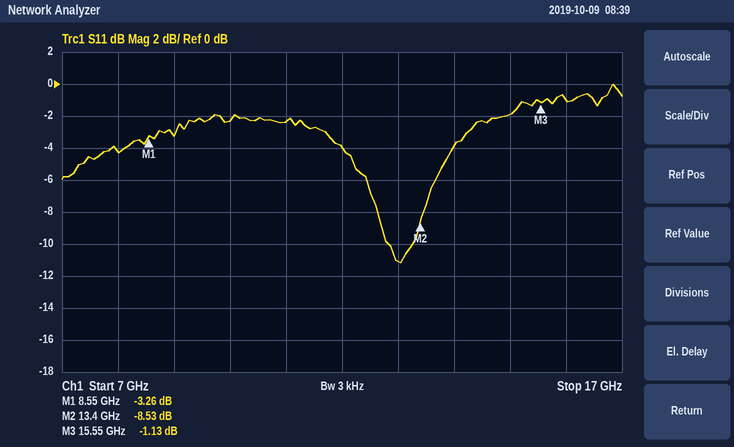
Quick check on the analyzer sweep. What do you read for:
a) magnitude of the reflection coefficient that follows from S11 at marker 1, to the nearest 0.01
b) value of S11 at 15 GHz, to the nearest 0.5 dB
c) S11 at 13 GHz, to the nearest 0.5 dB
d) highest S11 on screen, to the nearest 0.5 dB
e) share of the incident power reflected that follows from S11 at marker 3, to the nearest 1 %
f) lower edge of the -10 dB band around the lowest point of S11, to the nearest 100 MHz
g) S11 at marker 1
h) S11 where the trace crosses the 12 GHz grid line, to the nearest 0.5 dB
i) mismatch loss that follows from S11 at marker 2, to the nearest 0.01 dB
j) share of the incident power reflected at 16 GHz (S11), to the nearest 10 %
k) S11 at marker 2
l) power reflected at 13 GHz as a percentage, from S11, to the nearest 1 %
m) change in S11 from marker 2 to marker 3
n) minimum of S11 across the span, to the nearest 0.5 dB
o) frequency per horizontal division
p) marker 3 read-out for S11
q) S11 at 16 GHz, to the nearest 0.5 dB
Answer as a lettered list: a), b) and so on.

a) 0.69
b) -2.0 dB
c) -11.0 dB
d) 0.0 dB
e) 77 %
f) 12.8 GHz
g) -3.26 dB
h) -4.0 dB
i) 0.66 dB
j) 80 %
k) -8.53 dB
l) 8 %
m) 7.40 dB
n) -11.0 dB
o) 1 GHz
p) -1.13 dB
q) -1.0 dB
